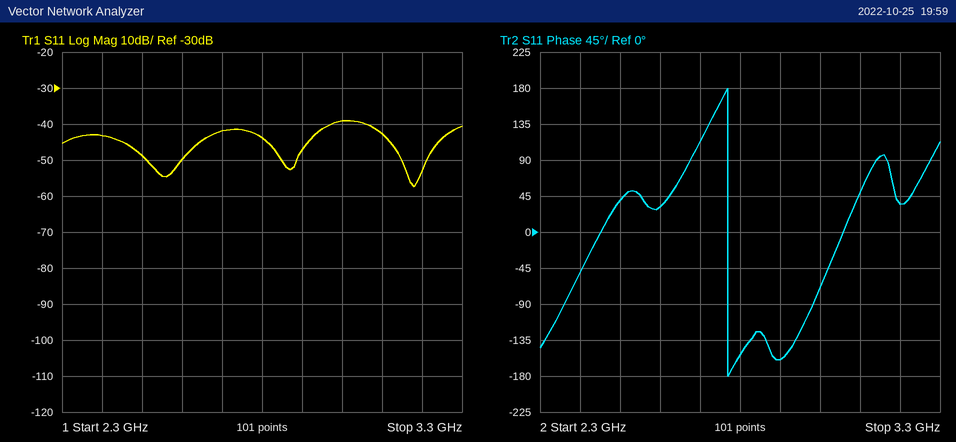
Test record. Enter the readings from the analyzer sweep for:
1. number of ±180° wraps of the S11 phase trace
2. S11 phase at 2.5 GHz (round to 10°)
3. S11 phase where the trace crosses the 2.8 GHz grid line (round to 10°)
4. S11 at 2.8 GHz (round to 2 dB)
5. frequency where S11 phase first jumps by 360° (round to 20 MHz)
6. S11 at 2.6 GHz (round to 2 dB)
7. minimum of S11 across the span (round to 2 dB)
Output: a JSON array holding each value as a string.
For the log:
["1", "40°", "-150°", "-44 dB", "2.76 GHz", "-50 dB", "-58 dB"]
